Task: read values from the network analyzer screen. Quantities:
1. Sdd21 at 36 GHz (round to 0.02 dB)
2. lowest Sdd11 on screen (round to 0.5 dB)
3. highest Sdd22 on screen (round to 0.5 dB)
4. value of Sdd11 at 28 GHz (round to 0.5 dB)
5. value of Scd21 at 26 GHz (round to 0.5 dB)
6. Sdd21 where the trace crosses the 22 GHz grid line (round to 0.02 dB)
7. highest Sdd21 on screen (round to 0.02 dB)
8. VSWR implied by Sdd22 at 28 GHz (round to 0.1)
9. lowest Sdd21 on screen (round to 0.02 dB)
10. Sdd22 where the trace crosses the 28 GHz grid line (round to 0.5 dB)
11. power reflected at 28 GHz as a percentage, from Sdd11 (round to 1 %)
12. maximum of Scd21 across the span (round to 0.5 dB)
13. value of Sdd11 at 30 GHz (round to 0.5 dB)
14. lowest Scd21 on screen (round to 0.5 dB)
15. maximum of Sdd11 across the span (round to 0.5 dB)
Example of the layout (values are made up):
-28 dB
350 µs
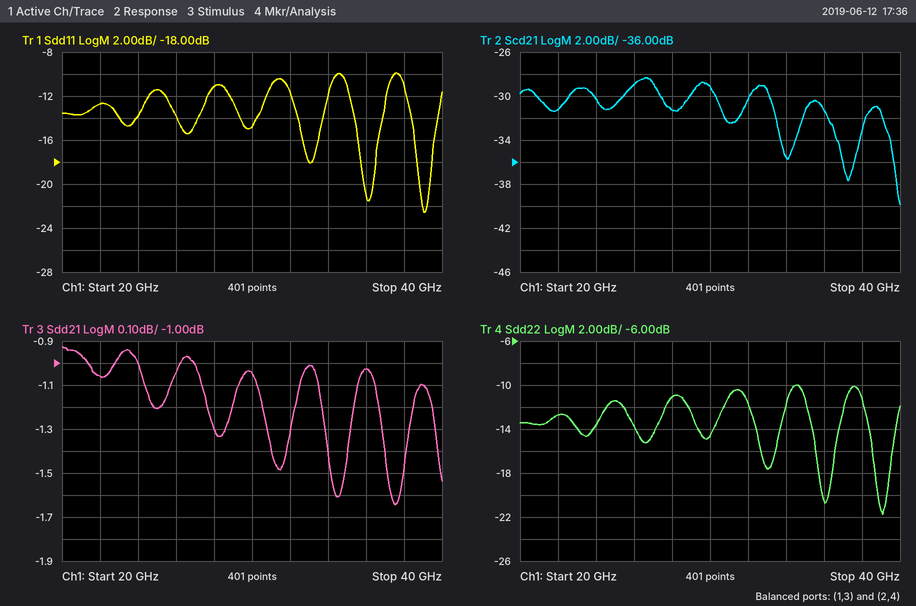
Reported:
-1.02 dB
-22.5 dB
-10.0 dB
-11.0 dB
-29.0 dB
-1.06 dB
-0.92 dB
1.8
-1.64 dB
-11.0 dB
8 %
-28.5 dB
-15.0 dB
-40.0 dB
-10.0 dB
